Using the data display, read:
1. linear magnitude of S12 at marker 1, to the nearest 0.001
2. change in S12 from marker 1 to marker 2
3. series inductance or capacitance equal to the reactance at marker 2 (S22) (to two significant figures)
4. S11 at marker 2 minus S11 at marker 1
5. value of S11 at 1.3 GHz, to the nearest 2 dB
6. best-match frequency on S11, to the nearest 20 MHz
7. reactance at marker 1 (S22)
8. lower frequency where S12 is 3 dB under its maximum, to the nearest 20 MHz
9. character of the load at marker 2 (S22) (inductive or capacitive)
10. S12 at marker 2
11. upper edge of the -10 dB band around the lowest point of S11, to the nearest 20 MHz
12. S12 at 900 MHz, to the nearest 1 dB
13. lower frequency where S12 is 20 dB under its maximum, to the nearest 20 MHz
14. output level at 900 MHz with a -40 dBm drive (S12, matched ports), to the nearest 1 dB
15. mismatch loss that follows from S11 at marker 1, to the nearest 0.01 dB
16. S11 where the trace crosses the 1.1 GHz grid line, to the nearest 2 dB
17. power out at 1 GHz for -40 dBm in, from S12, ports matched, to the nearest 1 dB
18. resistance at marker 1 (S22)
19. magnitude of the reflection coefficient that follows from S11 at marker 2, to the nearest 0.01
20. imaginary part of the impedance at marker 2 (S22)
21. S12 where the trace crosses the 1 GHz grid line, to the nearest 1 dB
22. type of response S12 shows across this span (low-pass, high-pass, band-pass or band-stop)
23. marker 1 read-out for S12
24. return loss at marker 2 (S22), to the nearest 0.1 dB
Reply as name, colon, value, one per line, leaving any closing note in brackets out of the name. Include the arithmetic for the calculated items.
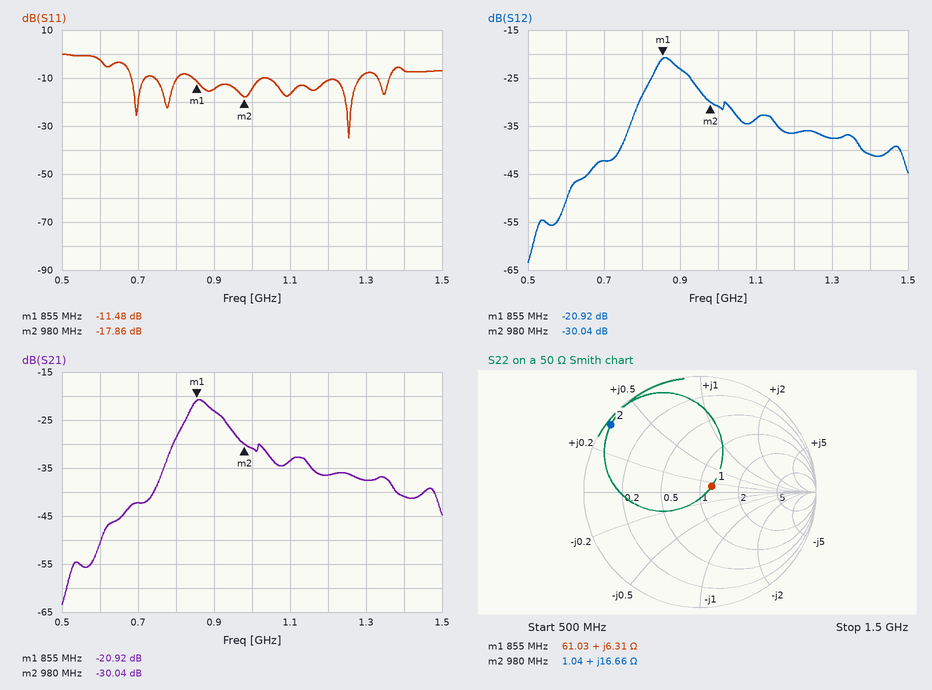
linear magnitude of S12 at marker 1, to the nearest 0.001: 10^(-20.92/20) ≈ 0.090
change in S12 from marker 1 to marker 2: -30.04 − (-20.92) = -9.12 dB
series inductance or capacitance equal to the reactance at marker 2 (S22): L = 16.66 Ω/(2π × 980 MHz) ≈ 2.7 nH
S11 at marker 2 minus S11 at marker 1: -17.86 − (-11.48) = -6.38 dB
value of S11 at 1.3 GHz, to the nearest 2 dB: -8 dB
best-match frequency on S11, to the nearest 20 MHz: 1.26 GHz
reactance at marker 1: +6.31 Ω
lower frequency where S12 is 3 dB under its maximum, to the nearest 20 MHz: 840 MHz
character of the load at marker 2 (S22): inductive
S12 at marker 2: -30.04 dB
upper edge of the -10 dB band around the lowest point of S11, to the nearest 20 MHz: 1.28 GHz
S12 at 900 MHz, to the nearest 1 dB: -23 dB
lower frequency where S12 is 20 dB under its maximum, to the nearest 20 MHz: 740 MHz
output level at 900 MHz with a -40 dBm drive (S12, matched ports), to the nearest 1 dB: -40 dBm + (-23 dB) = -63 dBm
mismatch loss that follows from S11 at marker 1, to the nearest 0.01 dB: −10 log10(1 − 10^(-11.48/10)) ≈ 0.32 dB
S11 where the trace crosses the 1.1 GHz grid line, to the nearest 2 dB: -16 dB
power out at 1 GHz for -40 dBm in, from S12, ports matched, to the nearest 1 dB: -40 dBm + (-31 dB) = -71 dBm
resistance at marker 1: 61.03 Ω
magnitude of the reflection coefficient that follows from S11 at marker 2, to the nearest 0.01: 10^(-17.86/20) ≈ 0.13
imaginary part of the impedance at marker 2: +16.66 Ω
S12 where the trace crosses the 1 GHz grid line, to the nearest 1 dB: -31 dB
type of response S12 shows across this span: band-pass
marker 1 read-out for S12: -20.92 dB
return loss at marker 2 (S22), to the nearest 0.1 dB: 0.3 dB
